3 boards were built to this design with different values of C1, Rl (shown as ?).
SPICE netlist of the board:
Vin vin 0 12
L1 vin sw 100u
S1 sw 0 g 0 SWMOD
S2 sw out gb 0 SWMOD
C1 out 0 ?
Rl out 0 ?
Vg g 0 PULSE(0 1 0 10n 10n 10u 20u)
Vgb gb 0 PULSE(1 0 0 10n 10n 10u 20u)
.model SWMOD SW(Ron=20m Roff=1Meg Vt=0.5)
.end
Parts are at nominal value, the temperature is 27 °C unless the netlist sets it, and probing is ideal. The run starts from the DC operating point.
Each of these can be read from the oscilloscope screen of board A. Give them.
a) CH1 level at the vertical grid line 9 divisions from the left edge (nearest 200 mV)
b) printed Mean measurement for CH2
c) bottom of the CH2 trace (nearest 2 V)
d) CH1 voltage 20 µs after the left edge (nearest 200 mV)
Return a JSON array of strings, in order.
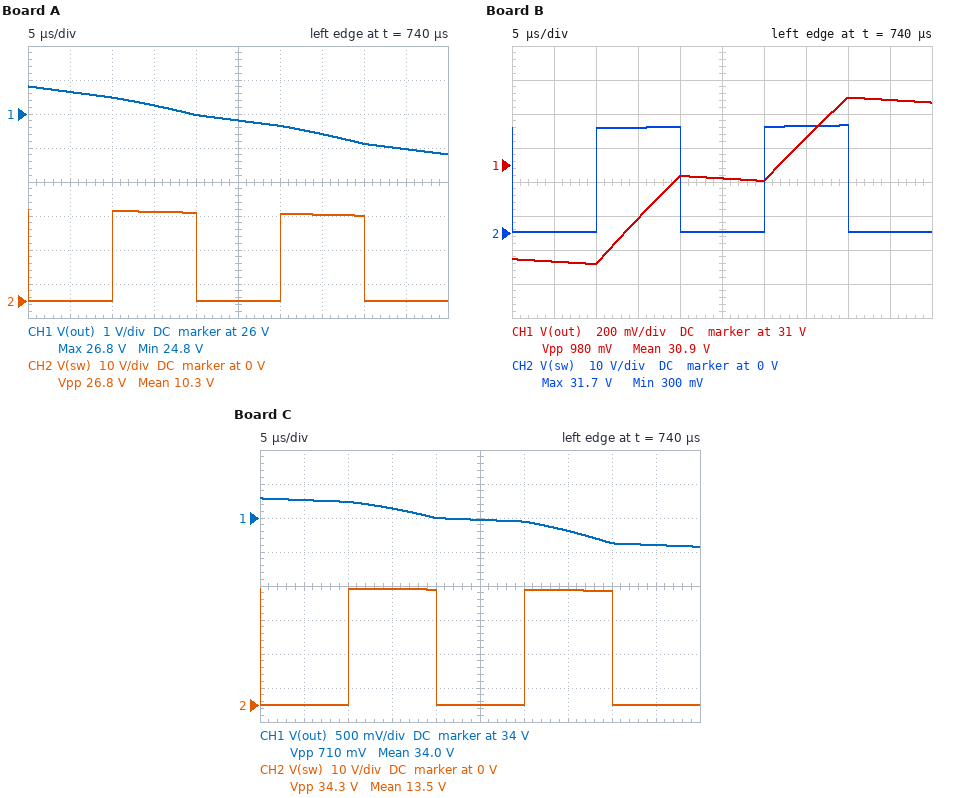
["25.0 V", "10.3 V", "0 V", "26.0 V"]
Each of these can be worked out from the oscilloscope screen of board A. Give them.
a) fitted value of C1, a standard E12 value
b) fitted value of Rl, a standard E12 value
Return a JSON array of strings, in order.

["68 µF", "12 Ω"]
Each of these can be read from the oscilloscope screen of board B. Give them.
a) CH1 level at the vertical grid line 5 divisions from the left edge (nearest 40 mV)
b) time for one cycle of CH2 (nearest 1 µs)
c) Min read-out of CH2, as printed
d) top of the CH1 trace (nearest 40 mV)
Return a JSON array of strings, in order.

["30.92 V", "20 µs", "300 mV", "31.40 V"]
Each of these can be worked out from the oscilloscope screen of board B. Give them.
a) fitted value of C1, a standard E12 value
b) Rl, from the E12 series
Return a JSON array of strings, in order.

["270 µF", "39 Ω"]
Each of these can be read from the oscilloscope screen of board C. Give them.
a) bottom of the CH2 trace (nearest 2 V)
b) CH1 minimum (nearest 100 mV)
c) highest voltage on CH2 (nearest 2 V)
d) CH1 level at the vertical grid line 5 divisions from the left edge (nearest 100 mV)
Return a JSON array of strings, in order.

["0 V", "33.6 V", "34 V", "34.0 V"]
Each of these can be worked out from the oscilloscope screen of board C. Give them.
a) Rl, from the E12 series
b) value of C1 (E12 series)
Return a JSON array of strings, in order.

["56 Ω", "120 µF"]
